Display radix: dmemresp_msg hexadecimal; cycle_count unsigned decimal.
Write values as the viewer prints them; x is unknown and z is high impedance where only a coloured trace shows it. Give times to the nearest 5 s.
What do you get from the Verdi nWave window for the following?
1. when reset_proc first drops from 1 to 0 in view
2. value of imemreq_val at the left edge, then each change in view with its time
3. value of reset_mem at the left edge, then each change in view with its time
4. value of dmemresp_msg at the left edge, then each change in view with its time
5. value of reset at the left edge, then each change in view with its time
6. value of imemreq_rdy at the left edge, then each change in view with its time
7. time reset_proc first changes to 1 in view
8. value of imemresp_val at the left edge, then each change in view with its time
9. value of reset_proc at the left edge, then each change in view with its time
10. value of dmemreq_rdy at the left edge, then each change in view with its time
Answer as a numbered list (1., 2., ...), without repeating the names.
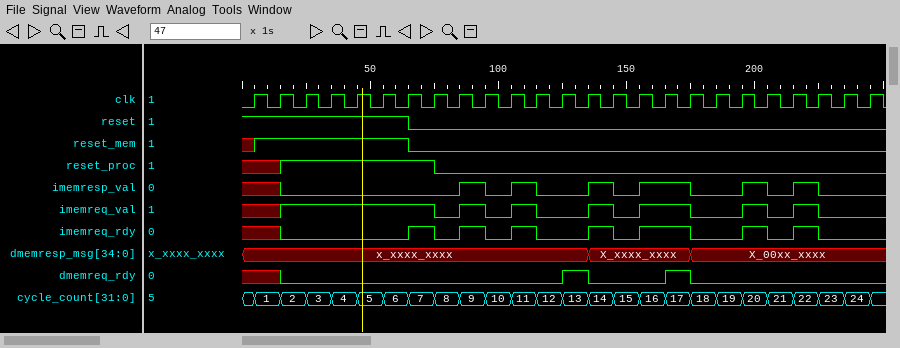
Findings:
1. 75 s
2. x, 1 at 15 s, 0 at 75 s, 1 at 85 s, 0 at 95 s, 1 at 105 s, 0 at 115 s, 1 at 135 s, 0 at 145 s, 1 at 155 s, 0 at 175 s, 1 at 195 s, 0 at 205 s, 1 at 215 s, 0 at 225 s
3. x, 1 at 5 s, 0 at 65 s
4. x_xxxx_xxxx, X_xxxx_xxxx at 135 s, X_00xx_xxxx at 175 s
5. 1, 0 at 65 s
6. x, 0 at 15 s, 1 at 65 s, 0 at 75 s, 1 at 85 s, 0 at 95 s, 1 at 105 s, 0 at 115 s, 1 at 135 s, 0 at 145 s, 1 at 155 s, 0 at 175 s, 1 at 195 s, 0 at 205 s, 1 at 215 s, 0 at 225 s
7. 15 s
8. x, 0 at 15 s, 1 at 85 s, 0 at 95 s, 1 at 105 s, 0 at 115 s, 1 at 135 s, 0 at 145 s, 1 at 155 s, 0 at 175 s, 1 at 195 s, 0 at 205 s, 1 at 215 s, 0 at 225 s
9. x, 1 at 15 s, 0 at 75 s
10. x, 0 at 15 s, 1 at 125 s, 0 at 135 s, 1 at 165 s, 0 at 175 s
